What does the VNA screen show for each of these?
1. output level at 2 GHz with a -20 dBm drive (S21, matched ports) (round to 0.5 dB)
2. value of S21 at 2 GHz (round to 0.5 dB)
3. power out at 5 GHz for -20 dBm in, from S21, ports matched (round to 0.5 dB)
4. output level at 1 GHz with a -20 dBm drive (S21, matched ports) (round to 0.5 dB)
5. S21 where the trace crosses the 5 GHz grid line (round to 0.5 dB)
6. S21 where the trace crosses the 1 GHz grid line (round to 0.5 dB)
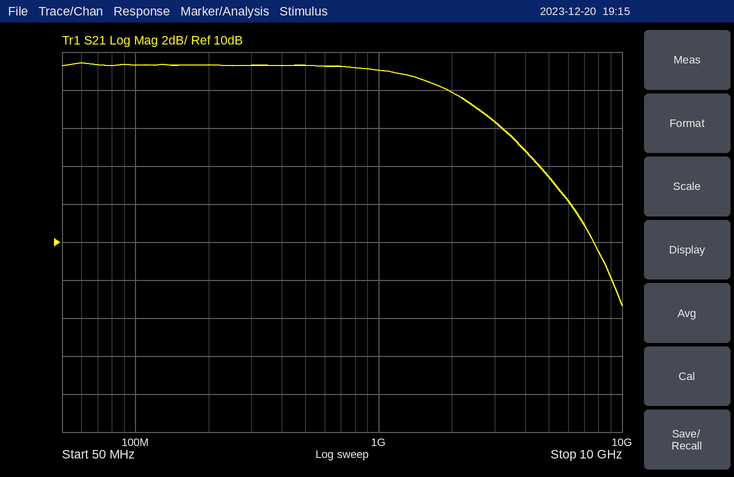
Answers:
-2.0 dBm
18.0 dB
-6.5 dBm
-1.0 dBm
13.5 dB
19.0 dB
